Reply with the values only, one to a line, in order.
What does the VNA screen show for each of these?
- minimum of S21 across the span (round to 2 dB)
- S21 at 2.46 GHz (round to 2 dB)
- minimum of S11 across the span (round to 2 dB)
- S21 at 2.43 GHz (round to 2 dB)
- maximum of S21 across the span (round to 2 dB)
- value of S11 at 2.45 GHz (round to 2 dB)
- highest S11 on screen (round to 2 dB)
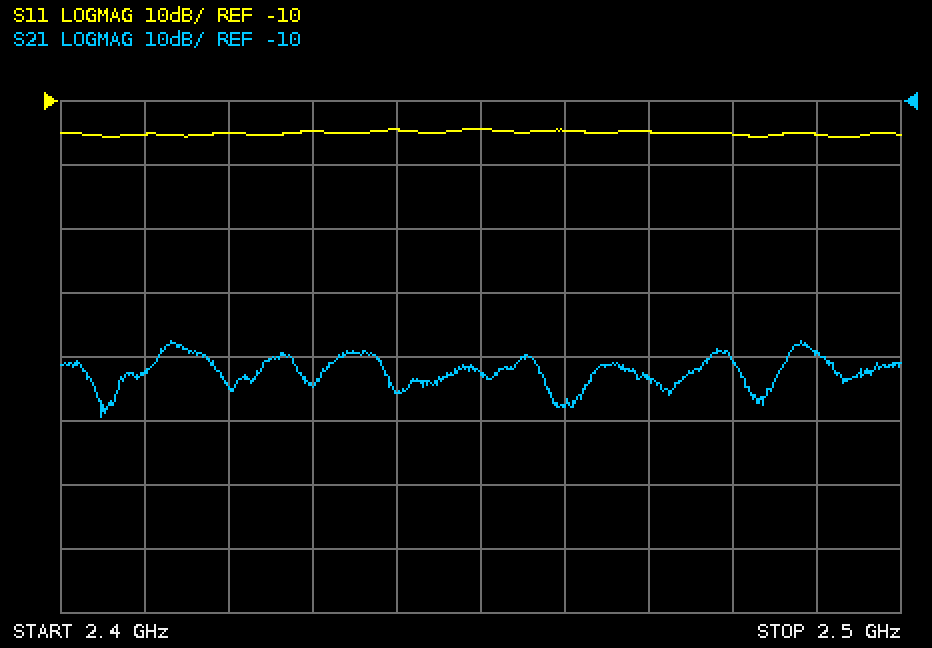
-60 dB
-58 dB
-16 dB
-54 dB
-48 dB
-14 dB
-14 dB
